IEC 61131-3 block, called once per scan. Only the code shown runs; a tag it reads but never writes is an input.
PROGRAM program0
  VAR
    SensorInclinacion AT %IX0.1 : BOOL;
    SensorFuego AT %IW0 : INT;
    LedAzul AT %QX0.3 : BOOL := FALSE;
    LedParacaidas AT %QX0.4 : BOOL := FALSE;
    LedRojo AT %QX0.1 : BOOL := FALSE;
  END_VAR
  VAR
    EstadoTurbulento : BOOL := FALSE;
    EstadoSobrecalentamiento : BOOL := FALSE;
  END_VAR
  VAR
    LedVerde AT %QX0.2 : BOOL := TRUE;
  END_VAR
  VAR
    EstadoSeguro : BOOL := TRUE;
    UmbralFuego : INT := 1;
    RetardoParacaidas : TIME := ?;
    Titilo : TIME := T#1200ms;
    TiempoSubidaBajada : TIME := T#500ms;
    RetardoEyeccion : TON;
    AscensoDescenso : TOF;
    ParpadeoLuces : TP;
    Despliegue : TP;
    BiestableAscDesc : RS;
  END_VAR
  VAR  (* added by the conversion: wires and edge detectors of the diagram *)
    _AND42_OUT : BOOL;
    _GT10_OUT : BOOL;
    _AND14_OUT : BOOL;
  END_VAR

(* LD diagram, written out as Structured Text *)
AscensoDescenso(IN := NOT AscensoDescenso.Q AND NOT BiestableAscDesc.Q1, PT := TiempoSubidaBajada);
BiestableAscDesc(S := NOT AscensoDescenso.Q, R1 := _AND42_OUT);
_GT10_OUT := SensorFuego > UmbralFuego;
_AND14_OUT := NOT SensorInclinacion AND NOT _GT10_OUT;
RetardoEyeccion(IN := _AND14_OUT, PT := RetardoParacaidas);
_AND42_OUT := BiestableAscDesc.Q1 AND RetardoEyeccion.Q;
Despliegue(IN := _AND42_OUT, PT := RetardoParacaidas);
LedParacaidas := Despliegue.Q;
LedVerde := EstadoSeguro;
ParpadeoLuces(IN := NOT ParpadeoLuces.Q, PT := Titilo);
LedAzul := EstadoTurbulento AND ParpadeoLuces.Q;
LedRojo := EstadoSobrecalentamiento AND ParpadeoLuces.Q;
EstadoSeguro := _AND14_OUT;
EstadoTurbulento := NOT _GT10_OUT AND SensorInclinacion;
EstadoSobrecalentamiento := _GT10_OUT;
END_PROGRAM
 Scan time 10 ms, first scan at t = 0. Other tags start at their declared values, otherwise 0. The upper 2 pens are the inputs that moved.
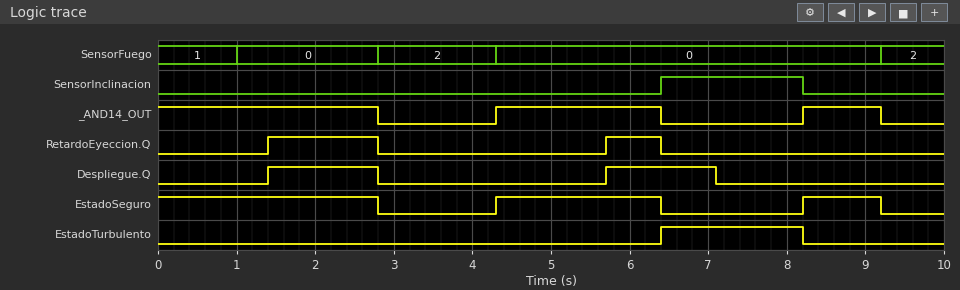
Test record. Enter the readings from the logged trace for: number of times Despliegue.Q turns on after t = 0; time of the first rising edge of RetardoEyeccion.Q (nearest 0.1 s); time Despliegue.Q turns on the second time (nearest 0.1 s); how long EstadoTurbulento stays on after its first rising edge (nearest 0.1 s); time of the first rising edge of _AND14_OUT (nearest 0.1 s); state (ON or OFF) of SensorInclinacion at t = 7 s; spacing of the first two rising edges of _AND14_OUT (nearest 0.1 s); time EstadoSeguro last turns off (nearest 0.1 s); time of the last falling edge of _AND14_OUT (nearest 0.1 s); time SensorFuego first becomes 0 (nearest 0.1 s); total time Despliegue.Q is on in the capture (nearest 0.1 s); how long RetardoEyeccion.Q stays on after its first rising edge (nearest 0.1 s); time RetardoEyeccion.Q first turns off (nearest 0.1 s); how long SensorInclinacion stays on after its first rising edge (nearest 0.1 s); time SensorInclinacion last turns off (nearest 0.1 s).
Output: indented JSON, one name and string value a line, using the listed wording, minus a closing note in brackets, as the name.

{
  "number of times Despliegue.Q turns on after t = 0": "2",
  "time of the first rising edge of RetardoEyeccion.Q": "1.4 s",
  "time Despliegue.Q turns on the second time": "5.7 s",
  "how long EstadoTurbulento stays on after its first rising edge": "1.8 s",
  "time of the first rising edge of _AND14_OUT": "4.3 s",
  "state (ON or OFF) of SensorInclinacion at t = 7 s": "ON",
  "spacing of the first two rising edges of _AND14_OUT": "3.9 s",
  "time EstadoSeguro last turns off": "9.2 s",
  "time of the last falling edge of _AND14_OUT": "9.2 s",
  "time SensorFuego first becomes 0": "1.0 s",
  "total time Despliegue.Q is on in the capture": "2.8 s",
  "how long RetardoEyeccion.Q stays on after its first rising edge": "1.4 s",
  "time RetardoEyeccion.Q first turns off": "2.8 s",
  "how long SensorInclinacion stays on after its first rising edge": "1.8 s",
  "time SensorInclinacion last turns off": "8.2 s"
}
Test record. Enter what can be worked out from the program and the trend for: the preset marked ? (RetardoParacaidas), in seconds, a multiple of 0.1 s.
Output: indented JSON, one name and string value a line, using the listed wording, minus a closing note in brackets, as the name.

{
  "the preset marked ? (RetardoParacaidas), in seconds, a multiple of 0.1 s": "1.4 s"
}
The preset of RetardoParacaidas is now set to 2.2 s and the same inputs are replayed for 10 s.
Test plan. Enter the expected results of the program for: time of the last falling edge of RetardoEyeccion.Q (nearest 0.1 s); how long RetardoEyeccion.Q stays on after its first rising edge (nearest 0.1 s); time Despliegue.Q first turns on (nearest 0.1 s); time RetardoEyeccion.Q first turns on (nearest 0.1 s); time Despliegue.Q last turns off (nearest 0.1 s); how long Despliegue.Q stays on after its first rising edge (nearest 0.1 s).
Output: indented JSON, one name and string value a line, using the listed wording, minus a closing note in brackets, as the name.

{
  "time of the last falling edge of RetardoEyeccion.Q": "2.8 s",
  "how long RetardoEyeccion.Q stays on after its first rising edge": "0.6 s",
  "time Despliegue.Q first turns on": "2.2 s",
  "time RetardoEyeccion.Q first turns on": "2.2 s",
  "time Despliegue.Q last turns off": "4.4 s",
  "how long Despliegue.Q stays on after its first rising edge": "2.2 s"
}
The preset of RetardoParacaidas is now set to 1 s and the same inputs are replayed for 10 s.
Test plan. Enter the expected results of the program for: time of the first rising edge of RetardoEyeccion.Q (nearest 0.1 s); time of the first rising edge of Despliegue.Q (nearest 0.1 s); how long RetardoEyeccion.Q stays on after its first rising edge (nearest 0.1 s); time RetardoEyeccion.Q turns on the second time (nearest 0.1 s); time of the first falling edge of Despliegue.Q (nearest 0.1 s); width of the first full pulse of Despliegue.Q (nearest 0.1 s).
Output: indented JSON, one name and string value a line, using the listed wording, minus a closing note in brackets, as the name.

{
  "time of the first rising edge of RetardoEyeccion.Q": "1.0 s",
  "time of the first rising edge of Despliegue.Q": "1.0 s",
  "how long RetardoEyeccion.Q stays on after its first rising edge": "1.8 s",
  "time RetardoEyeccion.Q turns on the second time": "5.3 s",
  "time of the first falling edge of Despliegue.Q": "2.0 s",
  "width of the first full pulse of Despliegue.Q": "1.0 s"
}
